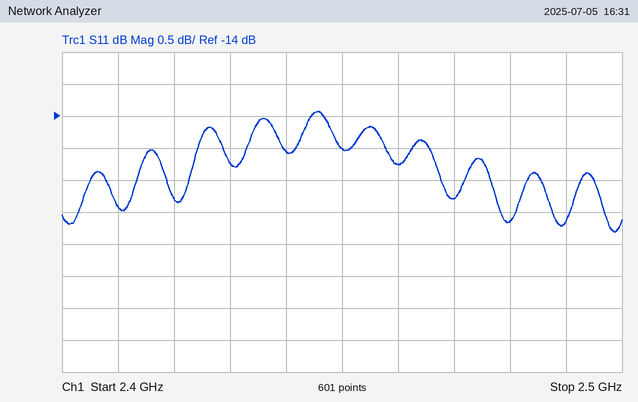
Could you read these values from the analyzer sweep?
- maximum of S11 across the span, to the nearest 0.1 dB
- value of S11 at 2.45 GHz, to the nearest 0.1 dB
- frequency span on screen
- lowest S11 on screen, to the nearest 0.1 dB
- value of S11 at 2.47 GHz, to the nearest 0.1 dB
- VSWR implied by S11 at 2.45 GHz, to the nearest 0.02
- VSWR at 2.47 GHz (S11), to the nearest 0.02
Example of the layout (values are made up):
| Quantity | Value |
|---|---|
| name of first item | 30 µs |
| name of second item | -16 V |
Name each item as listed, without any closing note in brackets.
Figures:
| Quantity | Value |
|---|---|
| maximum of S11 across the span, to the nearest 0.1 dB | -13.9 dB |
| value of S11 at 2.45 GHz, to the nearest 0.1 dB | -14.5 dB |
| frequency span on screen | 100 MHz |
| lowest S11 on screen, to the nearest 0.1 dB | -15.8 dB |
| value of S11 at 2.47 GHz, to the nearest 0.1 dB | -15.3 dB |
| VSWR implied by S11 at 2.45 GHz, to the nearest 0.02 | 1.46 |
| VSWR at 2.47 GHz (S11), to the nearest 0.02 | 1.42 |
